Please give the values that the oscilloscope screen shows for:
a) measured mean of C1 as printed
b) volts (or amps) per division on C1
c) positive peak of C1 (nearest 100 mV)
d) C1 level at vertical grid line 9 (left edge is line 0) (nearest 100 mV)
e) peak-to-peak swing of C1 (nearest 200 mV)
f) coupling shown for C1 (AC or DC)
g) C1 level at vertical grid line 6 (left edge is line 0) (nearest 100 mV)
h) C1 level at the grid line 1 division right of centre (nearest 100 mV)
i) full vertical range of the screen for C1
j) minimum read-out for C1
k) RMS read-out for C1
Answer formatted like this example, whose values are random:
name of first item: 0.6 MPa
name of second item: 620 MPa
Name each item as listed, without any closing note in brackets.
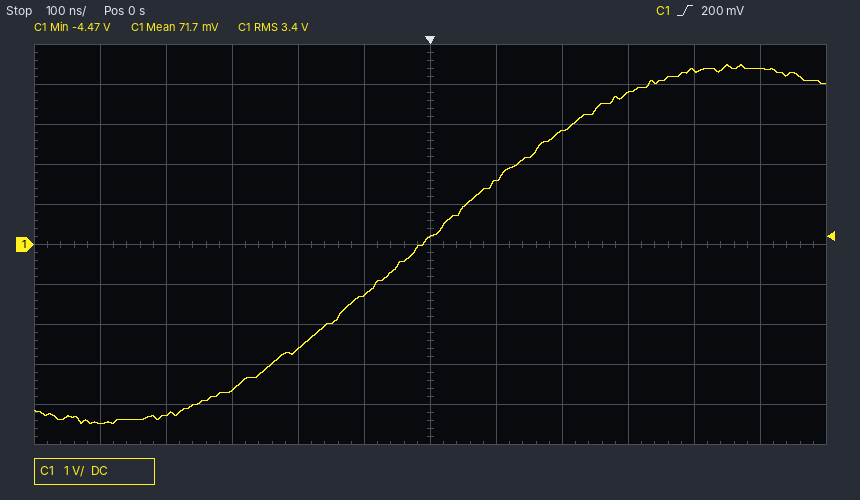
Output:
measured mean of C1 as printed: 71.7 mV
volts (or amps) per division on C1: 1 V
positive peak of C1: 4.5 V
C1 level at vertical grid line 9 (left edge is line 0): 3.8 V
peak-to-peak swing of C1: 9.0 V
coupling shown for C1: DC
C1 level at vertical grid line 6 (left edge is line 0): 200 mV
C1 level at the grid line 1 division right of centre: 1.6 V
full vertical range of the screen for C1: 10 V
minimum read-out for C1: -4.47 V
RMS read-out for C1: 3.4 V
